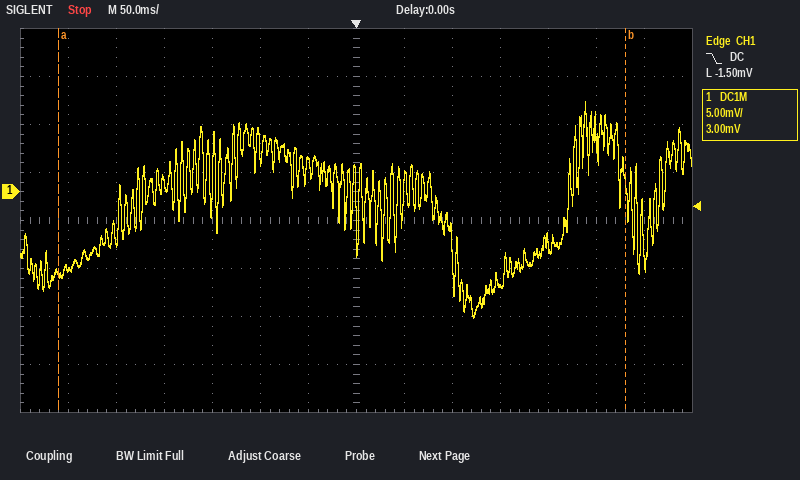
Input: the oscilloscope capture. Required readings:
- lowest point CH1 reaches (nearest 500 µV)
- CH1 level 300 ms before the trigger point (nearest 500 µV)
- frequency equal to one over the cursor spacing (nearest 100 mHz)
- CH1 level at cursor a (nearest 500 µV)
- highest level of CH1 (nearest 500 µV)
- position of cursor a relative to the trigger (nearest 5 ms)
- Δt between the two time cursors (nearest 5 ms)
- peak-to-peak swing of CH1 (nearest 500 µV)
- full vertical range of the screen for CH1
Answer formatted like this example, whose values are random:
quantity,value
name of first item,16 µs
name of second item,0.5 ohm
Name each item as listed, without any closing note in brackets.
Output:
quantity,value
lowest point CH1 reaches,-13.0 mV
CH1 level 300 ms before the trigger point,-8.0 mV
frequency equal to one over the cursor spacing,1.7 Hz
CH1 level at cursor a,-8.5 mV
highest level of CH1,9.5 mV
position of cursor a relative to the trigger,-310 ms
Δt between the two time cursors,590 ms
peak-to-peak swing of CH1,22.5 mV
full vertical range of the screen for CH1,40 mV
